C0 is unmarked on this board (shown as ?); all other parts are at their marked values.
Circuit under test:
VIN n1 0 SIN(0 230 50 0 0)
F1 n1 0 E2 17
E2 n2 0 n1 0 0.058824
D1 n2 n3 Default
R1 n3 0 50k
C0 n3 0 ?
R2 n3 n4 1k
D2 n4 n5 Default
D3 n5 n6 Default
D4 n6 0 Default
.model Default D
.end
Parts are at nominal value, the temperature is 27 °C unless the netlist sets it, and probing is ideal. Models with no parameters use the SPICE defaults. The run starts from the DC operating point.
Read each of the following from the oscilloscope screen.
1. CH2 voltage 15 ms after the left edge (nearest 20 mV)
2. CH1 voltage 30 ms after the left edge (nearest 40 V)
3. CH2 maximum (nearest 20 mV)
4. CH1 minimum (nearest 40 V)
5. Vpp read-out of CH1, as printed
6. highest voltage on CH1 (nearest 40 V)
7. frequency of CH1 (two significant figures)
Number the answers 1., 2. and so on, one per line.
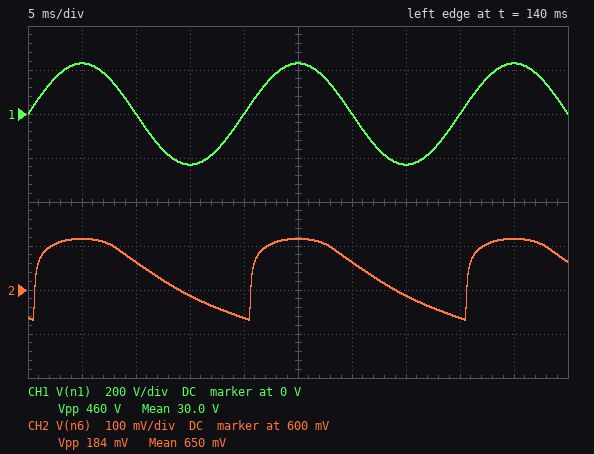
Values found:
1. 580 mV
2. 0 V
3. 720 mV
4. -240 V
5. 460 V
6. 240 V
7. 50 Hz
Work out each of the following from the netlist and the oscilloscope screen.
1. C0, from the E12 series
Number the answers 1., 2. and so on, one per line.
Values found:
1. 1.5 µF
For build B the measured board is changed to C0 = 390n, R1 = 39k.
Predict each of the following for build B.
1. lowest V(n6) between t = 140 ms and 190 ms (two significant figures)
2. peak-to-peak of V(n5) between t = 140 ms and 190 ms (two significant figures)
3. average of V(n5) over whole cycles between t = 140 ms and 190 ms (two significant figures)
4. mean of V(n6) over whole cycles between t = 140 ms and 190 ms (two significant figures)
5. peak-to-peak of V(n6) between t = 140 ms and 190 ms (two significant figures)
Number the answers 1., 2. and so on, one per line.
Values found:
1. 300 mV
2. 840 mV
3. 1.1 V
4. 550 mV
5. 420 mV
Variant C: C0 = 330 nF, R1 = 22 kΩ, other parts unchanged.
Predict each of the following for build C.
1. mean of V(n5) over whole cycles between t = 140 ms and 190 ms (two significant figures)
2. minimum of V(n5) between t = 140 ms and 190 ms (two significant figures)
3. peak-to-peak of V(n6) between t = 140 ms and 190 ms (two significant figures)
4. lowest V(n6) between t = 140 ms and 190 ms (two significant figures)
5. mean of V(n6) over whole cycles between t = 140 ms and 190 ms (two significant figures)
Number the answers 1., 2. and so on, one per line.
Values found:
1. 990 mV
2. 290 mV
3. 570 mV
4. 140 mV
5. 490 mV
